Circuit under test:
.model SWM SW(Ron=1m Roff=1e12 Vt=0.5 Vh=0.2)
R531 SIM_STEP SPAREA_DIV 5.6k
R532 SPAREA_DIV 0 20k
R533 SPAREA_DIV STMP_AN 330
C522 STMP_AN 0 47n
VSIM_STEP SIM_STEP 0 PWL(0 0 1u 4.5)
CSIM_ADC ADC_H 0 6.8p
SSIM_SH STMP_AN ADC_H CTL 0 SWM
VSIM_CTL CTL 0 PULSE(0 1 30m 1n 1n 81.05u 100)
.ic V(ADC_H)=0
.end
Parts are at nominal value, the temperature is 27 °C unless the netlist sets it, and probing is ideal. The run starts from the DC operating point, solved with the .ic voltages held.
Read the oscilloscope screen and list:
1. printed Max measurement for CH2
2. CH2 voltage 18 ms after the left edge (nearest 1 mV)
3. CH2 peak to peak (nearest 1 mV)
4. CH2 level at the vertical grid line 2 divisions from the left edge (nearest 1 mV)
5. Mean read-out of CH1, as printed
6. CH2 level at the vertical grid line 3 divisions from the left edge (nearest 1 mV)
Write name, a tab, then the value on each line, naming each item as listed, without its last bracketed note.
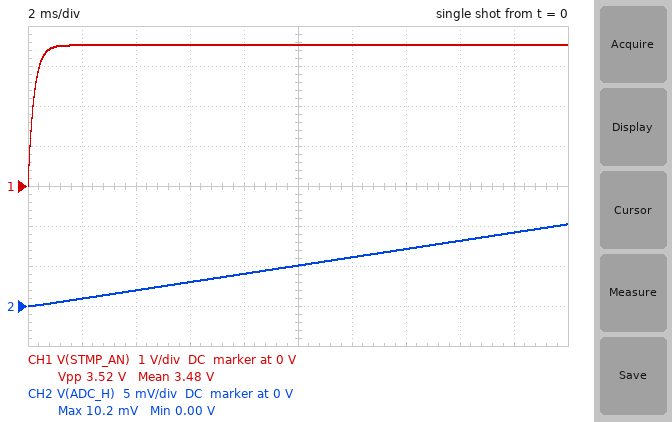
printed Max measurement for CH2	10.2 mV
CH2 voltage 18 ms after the left edge	9 mV
CH2 peak to peak	10 mV
CH2 level at the vertical grid line 2 divisions from the left edge	2 mV
Mean read-out of CH1, as printed	3.48 V
CH2 level at the vertical grid line 3 divisions from the left edge	3 mV
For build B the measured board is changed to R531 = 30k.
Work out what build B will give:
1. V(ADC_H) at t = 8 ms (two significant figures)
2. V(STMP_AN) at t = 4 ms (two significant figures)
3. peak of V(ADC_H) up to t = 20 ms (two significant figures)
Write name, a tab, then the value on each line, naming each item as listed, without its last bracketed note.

V(ADC_H) at t = 8 ms	2.0 mV
V(STMP_AN) at t = 4 ms	1.8 V
peak of V(ADC_H) up to t = 20 ms	5.1 mV
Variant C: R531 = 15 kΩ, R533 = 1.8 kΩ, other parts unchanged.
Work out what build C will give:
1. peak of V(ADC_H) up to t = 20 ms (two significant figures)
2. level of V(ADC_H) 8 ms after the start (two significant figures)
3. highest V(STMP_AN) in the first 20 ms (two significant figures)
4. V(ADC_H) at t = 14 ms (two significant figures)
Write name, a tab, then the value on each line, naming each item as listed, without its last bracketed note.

peak of V(ADC_H) up to t = 20 ms	7.4 mV
level of V(ADC_H) 8 ms after the start	2.8 mV
highest V(STMP_AN) in the first 20 ms	2.6 V
V(ADC_H) at t = 14 ms	5.1 mV
